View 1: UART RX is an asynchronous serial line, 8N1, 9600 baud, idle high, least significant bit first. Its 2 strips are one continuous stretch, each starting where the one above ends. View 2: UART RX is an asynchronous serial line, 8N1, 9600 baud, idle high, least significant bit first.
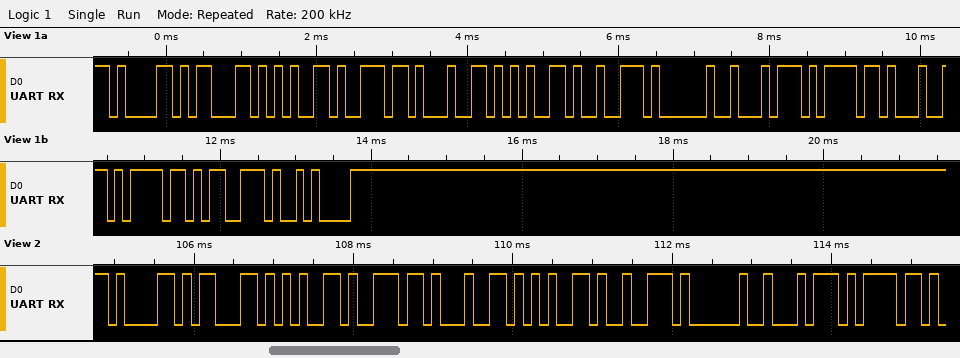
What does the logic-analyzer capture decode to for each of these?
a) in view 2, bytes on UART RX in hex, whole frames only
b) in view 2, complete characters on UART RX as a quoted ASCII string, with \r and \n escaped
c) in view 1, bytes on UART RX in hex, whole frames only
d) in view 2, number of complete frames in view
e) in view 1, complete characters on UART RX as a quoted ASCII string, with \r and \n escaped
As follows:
0x61 0x63 0x65 0x6E 0x64 0x65 0x72 0x20 0x74 0x6F
"acender to"
61 63 65 6E 64 65 72 20 74 6F 64 6F 73 0A
10
"acender todos\n"
